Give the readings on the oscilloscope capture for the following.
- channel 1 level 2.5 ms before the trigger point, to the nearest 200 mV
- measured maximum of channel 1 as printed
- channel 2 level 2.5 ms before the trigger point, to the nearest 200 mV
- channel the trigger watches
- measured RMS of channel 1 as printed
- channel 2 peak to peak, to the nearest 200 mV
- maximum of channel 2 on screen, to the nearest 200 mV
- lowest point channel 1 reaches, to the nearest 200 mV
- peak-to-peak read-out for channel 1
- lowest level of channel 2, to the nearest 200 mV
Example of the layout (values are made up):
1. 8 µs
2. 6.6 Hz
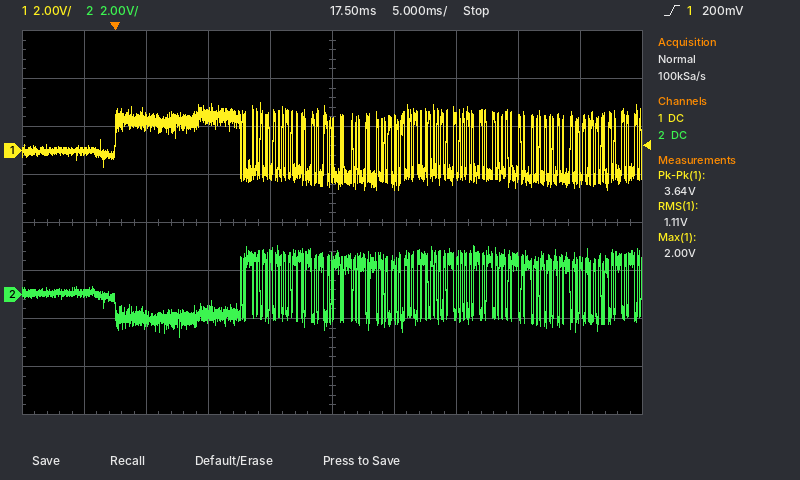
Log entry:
1. 0.0 V
2. 2.00 V
3. 0.0 V
4. channel 1
5. 1.11 V
6. 3.8 V
7. 2.0 V
8. -1.6 V
9. 3.64 V
10. -1.8 V
